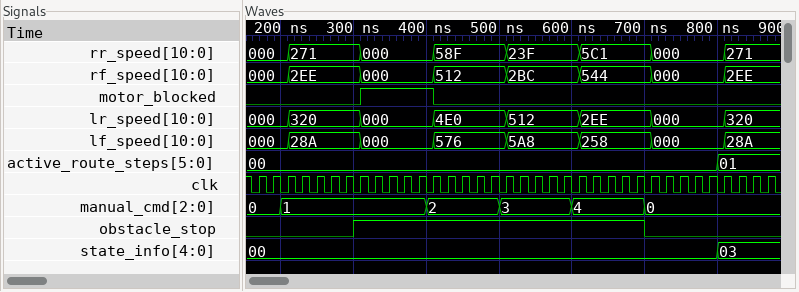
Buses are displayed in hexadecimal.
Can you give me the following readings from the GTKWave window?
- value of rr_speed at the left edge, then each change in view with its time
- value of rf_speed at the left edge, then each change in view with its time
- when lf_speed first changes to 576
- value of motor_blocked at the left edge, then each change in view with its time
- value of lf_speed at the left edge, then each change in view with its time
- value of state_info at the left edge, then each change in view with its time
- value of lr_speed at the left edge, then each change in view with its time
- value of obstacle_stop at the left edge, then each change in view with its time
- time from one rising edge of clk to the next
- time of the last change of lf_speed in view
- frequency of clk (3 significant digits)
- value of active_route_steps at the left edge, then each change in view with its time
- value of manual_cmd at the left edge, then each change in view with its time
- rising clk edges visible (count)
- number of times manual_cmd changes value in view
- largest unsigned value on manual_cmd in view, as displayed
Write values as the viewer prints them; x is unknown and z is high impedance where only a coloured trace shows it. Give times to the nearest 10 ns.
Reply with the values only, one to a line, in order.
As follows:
000, 271 at 210 ns, 000 at 310 ns, 58F at 410 ns, 23F at 510 ns, 5C1 at 610 ns, 000 at 710 ns, 271 at 810 ns
000, 2EE at 210 ns, 000 at 310 ns, 512 at 410 ns, 2BC at 510 ns, 544 at 610 ns, 000 at 710 ns, 2EE at 810 ns
410 ns
0, 1 at 310 ns, 0 at 410 ns
000, 28A at 210 ns, 000 at 310 ns, 576 at 410 ns, 5A8 at 510 ns, 258 at 610 ns, 000 at 710 ns, 28A at 810 ns
00, 03 at 800 ns
000, 320 at 210 ns, 000 at 310 ns, 4E0 at 410 ns, 512 at 510 ns, 2EE at 610 ns, 000 at 710 ns, 320 at 810 ns
0, 1 at 300 ns, 0 at 700 ns
20 ns
810 ns
50.0 MHz
00, 01 at 800 ns
0, 1 at 200 ns, 2 at 400 ns, 3 at 500 ns, 4 at 600 ns, 0 at 700 ns
36
5
4
